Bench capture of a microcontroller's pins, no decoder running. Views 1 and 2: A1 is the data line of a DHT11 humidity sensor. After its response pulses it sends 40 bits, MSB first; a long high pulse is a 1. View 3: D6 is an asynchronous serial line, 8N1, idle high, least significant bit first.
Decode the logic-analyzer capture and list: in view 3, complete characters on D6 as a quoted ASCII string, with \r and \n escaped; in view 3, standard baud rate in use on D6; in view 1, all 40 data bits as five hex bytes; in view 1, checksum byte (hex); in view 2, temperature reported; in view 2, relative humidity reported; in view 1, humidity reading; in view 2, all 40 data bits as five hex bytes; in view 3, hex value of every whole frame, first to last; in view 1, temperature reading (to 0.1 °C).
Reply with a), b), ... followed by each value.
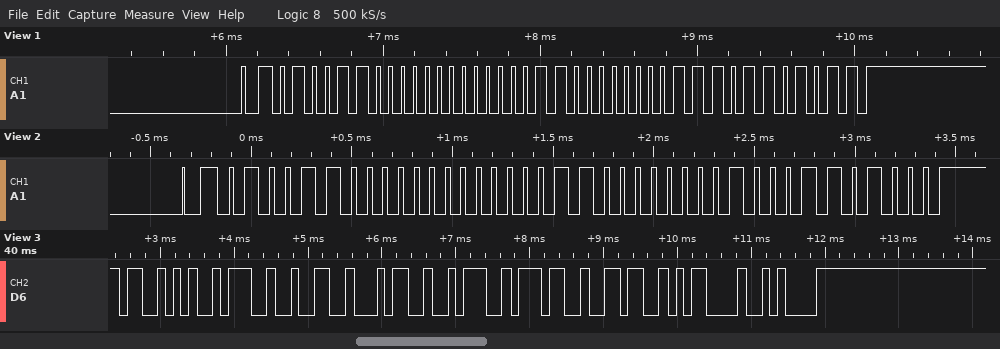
a) "S:24:76\r\n"
b) 9600 baud
c) 4C 00 18 07 6B
d) 0x6B
e) 24.4 °C
f) 76 %
g) 76 %
h) 4C 00 18 04 68
i) 53 3A 32 34 3A 37 36 0D 0A
j) 24.7 °C
